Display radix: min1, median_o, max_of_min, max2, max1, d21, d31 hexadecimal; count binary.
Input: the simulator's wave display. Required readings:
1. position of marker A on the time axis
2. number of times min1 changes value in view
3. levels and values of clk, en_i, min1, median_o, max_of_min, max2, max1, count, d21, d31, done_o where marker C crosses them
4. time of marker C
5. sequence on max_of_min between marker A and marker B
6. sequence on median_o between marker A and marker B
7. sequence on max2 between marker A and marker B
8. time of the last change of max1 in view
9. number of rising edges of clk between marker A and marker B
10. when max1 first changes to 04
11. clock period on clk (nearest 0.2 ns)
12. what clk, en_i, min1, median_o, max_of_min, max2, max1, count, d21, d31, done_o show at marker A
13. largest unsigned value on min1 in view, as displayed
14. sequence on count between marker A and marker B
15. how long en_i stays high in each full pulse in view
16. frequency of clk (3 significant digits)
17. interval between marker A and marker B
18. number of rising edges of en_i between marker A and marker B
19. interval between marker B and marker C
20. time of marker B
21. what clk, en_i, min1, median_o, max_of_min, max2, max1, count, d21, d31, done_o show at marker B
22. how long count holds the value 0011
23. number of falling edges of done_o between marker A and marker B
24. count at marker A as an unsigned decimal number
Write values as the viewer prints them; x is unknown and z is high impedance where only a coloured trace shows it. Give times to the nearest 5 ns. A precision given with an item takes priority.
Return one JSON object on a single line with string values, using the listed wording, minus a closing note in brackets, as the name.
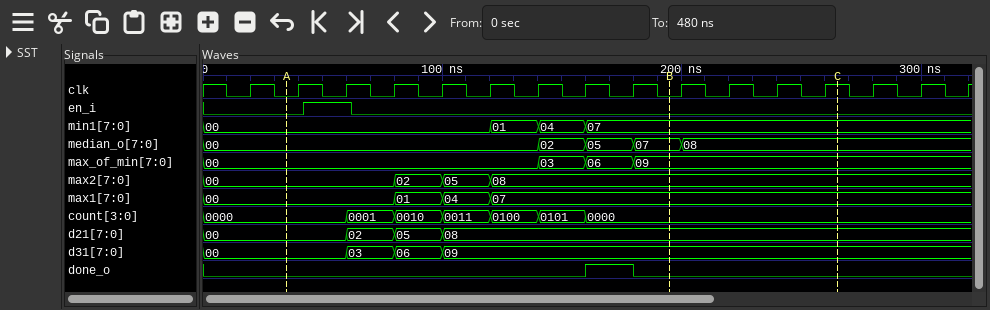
{"position of marker A on the time axis": "35 ns", "number of times min1 changes value in view": "3", "levels and values of clk, en_i, min1, median_o, max_of_min, max2, max1, count, d21, d31, done_o where marker C crosses them": "clk=1, en_i=0, min1=07, median_o=08, max_of_min=09, max2=08, max1=07, count=0000, d21=08, d31=09, done_o=0", "time of marker C": "265 ns", "sequence on max_of_min between marker A and marker B": "00, 03, 06, 09", "sequence on median_o between marker A and marker B": "00, 02, 05, 07", "sequence on max2 between marker A and marker B": "00, 02, 05, 08", "time of the last change of max1 in view": "120 ns", "number of rising edges of clk between marker A and marker B": "8", "when max1 first changes to 04": "100 ns", "clock period on clk": "20 ns", "what clk, en_i, min1, median_o, max_of_min, max2, max1, count, d21, d31, done_o show at marker A": "clk=0, en_i=0, min1=00, median_o=00, max_of_min=00, max2=00, max1=00, count=0000, d21=00, d31=00, done_o=0", "largest unsigned value on min1 in view, as displayed": "07", "sequence on count between marker A and marker B": "0000, 0001, 0010, 0011, 0100, 0101, 0000", "how long en_i stays high in each full pulse in view": "20 ns", "frequency of clk": "50.0 MHz", "interval between marker A and marker B": "160 ns", "number of rising edges of en_i between marker A and marker B": "1", "interval between marker B and marker C": "70 ns", "time of marker B": "195 ns", "what clk, en_i, min1, median_o, max_of_min, max2, max1, count, d21, d31, done_o show at marker B": "clk=0, en_i=0, min1=07, median_o=07, max_of_min=09, max2=08, max1=07, count=0000, d21=08, d31=09, done_o=0", "how long count holds the value 0011": "20 ns", "number of falling edges of done_o between marker A and marker B": "1", "count at marker A as an unsigned decimal number": "0"}
